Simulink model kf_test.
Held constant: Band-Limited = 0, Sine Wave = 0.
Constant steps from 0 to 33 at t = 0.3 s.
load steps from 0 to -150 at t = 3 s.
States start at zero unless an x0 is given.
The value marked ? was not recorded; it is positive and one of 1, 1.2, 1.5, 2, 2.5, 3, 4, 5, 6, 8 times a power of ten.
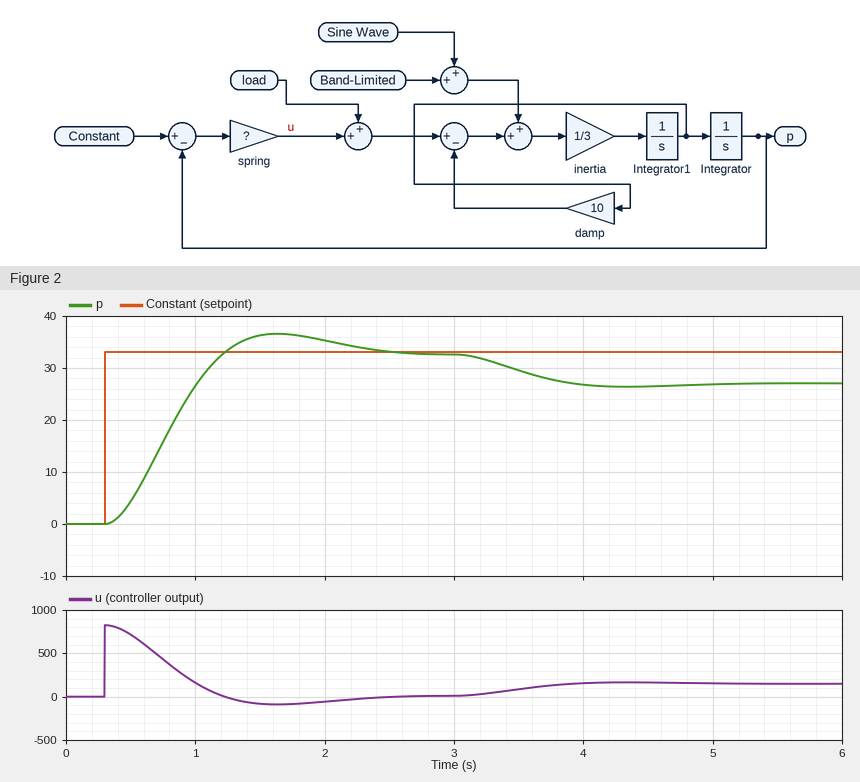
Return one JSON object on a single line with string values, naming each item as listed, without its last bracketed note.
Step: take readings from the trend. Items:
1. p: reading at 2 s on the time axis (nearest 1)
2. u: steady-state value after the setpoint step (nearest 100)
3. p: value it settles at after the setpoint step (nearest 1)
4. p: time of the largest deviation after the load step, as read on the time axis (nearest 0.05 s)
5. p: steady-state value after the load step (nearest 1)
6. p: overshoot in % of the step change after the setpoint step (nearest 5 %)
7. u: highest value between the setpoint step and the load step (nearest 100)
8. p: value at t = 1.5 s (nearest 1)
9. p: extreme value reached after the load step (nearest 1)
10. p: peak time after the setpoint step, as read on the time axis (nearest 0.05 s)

{"p: reading at 2 s on the time axis": "35", "u: steady-state value after the setpoint step": "0", "p: value it settles at after the setpoint step": "33", "p: time of the largest deviation after the load step, as read on the time axis": "4.35 s", "p: steady-state value after the load step": "27", "p: overshoot in % of the step change after the setpoint step": "10 %", "u: highest value between the setpoint step and the load step": "800", "p: value at t = 1.5 s": "36", "p: extreme value reached after the load step": "26", "p: peak time after the setpoint step, as read on the time axis": "1.65 s"}
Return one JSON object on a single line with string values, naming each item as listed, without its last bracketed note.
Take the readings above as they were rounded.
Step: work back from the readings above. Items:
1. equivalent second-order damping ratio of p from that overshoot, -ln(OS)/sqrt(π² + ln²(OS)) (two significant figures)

{"equivalent second-order damping ratio of p from that overshoot, -ln(OS)/sqrt(π² + ln²(OS))": "0.59"}
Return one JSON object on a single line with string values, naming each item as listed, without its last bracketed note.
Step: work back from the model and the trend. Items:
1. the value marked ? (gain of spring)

{"the value marked ?": "25"}
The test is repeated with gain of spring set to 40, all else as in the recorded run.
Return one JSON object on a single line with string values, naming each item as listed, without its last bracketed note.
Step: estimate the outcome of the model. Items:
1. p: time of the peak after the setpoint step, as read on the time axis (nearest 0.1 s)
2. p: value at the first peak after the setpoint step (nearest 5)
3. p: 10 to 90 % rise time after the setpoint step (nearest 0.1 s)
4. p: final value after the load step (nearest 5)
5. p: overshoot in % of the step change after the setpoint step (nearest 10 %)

{"p: time of the peak after the setpoint step, as read on the time axis": "1.3 s", "p: value at the first peak after the setpoint step": "40", "p: 10 to 90 % rise time after the setpoint step": "0.4 s", "p: final value after the load step": "30", "p: overshoot in % of the step change after the setpoint step": "20 %"}
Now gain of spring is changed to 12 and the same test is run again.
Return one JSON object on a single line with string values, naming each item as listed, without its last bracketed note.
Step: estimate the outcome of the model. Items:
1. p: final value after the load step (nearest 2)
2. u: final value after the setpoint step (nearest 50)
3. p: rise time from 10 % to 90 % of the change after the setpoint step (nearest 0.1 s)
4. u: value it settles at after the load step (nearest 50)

{"p: final value after the load step": "20", "u: final value after the setpoint step": "0", "p: rise time from 10 % to 90 % of the change after the setpoint step": "1.3 s", "u: value it settles at after the load step": "150"}
